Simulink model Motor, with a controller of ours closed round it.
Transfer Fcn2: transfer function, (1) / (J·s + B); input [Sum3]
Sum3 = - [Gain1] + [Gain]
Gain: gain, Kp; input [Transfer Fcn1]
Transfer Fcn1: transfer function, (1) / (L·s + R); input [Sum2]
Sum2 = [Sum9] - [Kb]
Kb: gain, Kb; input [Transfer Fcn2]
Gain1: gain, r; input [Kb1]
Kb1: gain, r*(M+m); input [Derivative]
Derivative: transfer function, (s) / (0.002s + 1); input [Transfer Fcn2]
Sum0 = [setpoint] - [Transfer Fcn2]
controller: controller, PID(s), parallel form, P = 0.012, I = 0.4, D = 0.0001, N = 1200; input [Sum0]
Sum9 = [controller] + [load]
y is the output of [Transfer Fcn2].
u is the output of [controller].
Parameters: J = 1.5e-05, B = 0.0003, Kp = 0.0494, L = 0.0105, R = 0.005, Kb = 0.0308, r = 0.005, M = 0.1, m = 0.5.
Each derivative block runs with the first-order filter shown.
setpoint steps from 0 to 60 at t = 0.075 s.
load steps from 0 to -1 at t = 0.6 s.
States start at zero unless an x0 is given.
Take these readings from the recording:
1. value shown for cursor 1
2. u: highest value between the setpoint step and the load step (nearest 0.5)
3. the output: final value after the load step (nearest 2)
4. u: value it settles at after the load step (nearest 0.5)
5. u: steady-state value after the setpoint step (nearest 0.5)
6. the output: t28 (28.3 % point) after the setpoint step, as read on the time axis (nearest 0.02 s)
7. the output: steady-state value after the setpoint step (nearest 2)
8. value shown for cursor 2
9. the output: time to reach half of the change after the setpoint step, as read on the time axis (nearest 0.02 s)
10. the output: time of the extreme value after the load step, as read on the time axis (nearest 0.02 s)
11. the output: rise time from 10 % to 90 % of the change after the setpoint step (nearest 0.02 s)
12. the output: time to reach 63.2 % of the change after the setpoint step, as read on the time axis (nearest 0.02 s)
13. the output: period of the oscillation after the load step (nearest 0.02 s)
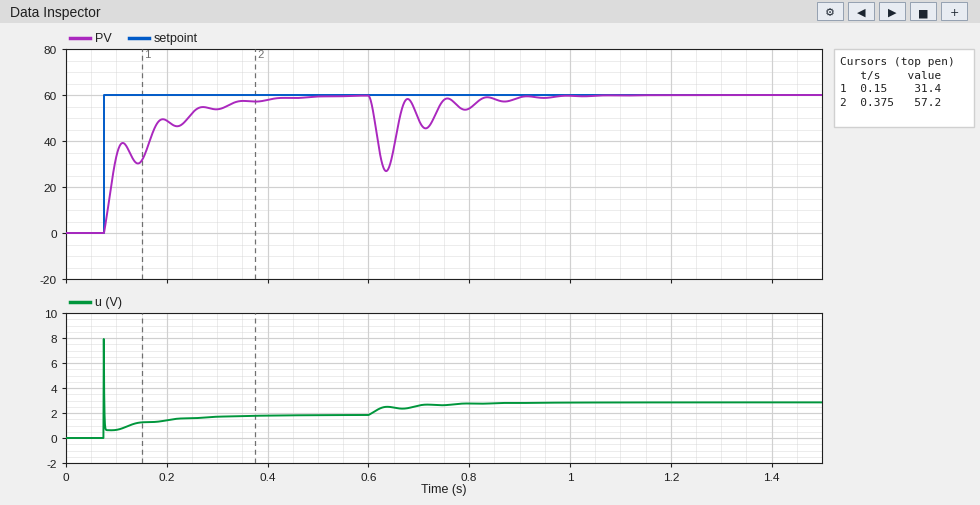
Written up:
31.4
8.0
60
3.0
2.0
0.08 s
60
57.2
0.10 s
0.64 s
0.18 s
0.10 s
0.08 s
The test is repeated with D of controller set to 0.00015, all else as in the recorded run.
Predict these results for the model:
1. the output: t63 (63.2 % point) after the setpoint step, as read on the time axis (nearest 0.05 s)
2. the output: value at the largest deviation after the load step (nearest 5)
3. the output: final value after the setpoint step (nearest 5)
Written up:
0.15 s
30
60
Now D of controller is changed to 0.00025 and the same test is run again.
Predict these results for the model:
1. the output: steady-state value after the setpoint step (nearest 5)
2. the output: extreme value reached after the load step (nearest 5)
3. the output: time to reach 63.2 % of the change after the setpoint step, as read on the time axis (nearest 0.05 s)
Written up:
60
30
0.15 s
